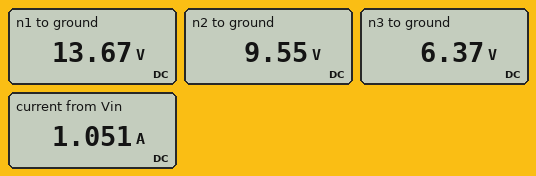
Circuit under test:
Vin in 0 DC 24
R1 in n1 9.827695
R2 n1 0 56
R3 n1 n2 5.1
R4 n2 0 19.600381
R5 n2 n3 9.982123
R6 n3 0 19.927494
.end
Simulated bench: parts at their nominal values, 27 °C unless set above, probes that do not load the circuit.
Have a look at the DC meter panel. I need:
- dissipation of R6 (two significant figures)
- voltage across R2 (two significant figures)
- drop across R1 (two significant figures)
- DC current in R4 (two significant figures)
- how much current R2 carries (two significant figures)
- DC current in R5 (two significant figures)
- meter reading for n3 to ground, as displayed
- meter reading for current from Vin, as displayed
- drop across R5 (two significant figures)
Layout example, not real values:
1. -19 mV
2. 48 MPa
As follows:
1. 2.0 W
2. 14 V
3. 10 V
4. 490 mA
5. 240 mA
6. 320 mA
7. 6.37 V
8. 1.051 A
9. 3.2 V
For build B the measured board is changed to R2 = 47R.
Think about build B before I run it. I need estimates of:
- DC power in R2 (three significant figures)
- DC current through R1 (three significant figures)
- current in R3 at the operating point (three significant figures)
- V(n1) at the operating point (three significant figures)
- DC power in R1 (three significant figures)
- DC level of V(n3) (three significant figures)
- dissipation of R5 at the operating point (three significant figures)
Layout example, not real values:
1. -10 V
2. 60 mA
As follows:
1. 3.83 W
2. 1.08 A
3. 792 mA
4. 13.4 V
5. 11.4 W
6. 6.25 V
7. 981 mW
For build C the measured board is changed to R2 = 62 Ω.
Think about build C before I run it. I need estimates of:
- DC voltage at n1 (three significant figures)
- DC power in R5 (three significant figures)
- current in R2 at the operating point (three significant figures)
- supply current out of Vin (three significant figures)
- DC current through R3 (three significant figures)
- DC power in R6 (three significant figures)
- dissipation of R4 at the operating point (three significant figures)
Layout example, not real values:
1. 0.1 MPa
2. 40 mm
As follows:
1. 13.8 V
2. 1.04 W
3. 223 mA
4. 1.04 A
5. 815 mA
6. 2.07 W
7. 4.75 W
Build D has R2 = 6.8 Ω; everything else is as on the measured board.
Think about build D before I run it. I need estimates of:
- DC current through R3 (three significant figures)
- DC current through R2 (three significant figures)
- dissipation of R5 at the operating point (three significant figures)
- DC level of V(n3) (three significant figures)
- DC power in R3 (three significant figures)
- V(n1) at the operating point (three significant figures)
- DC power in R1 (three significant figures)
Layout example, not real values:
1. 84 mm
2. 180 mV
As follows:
1. 468 mA
2. 1.17 A
3. 343 mW
4. 3.69 V
5. 1.12 W
6. 7.93 V
7. 26.3 W
